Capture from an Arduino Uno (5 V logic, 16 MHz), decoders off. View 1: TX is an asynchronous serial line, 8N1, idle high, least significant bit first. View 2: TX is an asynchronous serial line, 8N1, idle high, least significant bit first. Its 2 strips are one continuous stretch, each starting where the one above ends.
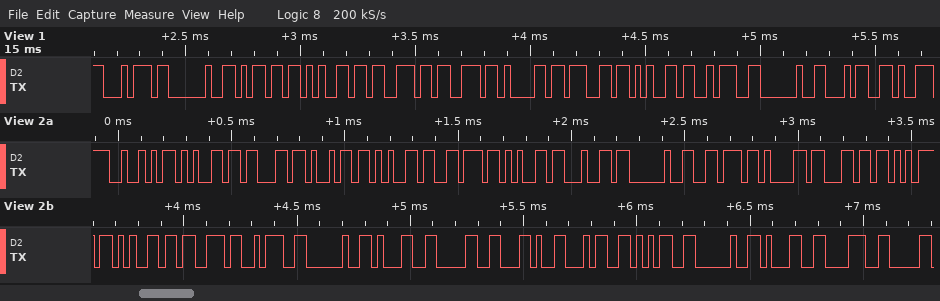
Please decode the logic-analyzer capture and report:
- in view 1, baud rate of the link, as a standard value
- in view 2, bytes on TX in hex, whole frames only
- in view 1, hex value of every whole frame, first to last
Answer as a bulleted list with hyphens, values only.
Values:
- 38400 baud
- 0x52 0x65 0x63 0x69 0x65 0x76 0x65 0x64 0x20 0x76 0x61 0x6C 0x75 0x65 0x73 0x3A 0x20 0x31 0x30 0x2C 0x34 0x35 0x20 0x31 0x38
- 74 20 6D 65 73 73 61 67 65 3A 20 34
